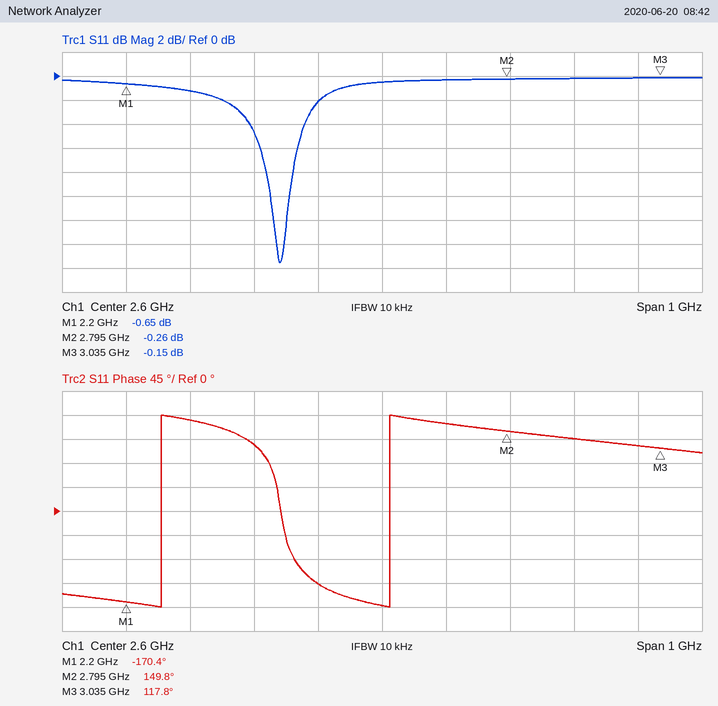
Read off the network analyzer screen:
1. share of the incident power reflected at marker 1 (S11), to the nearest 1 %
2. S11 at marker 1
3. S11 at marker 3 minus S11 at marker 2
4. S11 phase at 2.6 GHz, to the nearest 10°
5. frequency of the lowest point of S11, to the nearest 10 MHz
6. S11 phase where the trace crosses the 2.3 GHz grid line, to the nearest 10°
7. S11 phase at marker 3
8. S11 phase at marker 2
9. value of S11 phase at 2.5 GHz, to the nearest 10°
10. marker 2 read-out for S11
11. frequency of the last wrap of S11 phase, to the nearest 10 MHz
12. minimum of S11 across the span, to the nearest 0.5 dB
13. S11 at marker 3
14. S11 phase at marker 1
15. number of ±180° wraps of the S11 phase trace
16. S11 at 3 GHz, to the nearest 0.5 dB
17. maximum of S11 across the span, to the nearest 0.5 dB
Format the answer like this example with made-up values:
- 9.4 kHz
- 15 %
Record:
- 86 %
- -0.65 dB
- 0.11 dB
- -180°
- 2.44 GHz
- 170°
- 117.8°
- 149.8°
- -140°
- -0.26 dB
- 2.61 GHz
- -15.5 dB
- -0.15 dB
- -170.4°
- 2
- 0.0 dB
- 0.0 dB
